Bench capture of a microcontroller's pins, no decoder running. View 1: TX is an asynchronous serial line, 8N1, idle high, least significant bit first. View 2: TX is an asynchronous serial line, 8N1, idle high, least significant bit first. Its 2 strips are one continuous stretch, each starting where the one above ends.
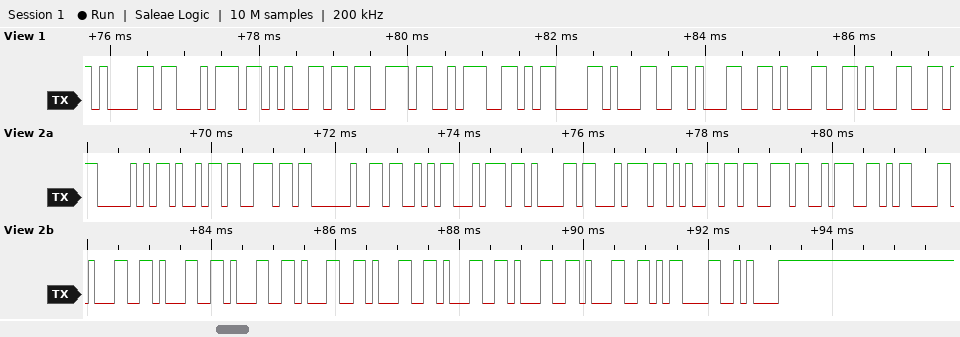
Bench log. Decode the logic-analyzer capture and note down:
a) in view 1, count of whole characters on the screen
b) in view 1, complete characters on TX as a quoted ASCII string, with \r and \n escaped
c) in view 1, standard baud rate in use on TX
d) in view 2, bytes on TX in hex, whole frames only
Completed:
10
"ates:\r1111"
9600 baud
0x50 0x69 0x6E 0x20 0x53 0x74 0x61 0x74 0x65 0x73 0x3A 0x0D 0x31 0x31 0x31 0x31 0x31 0x31 0x31 0x31 0x0D 0x0A
